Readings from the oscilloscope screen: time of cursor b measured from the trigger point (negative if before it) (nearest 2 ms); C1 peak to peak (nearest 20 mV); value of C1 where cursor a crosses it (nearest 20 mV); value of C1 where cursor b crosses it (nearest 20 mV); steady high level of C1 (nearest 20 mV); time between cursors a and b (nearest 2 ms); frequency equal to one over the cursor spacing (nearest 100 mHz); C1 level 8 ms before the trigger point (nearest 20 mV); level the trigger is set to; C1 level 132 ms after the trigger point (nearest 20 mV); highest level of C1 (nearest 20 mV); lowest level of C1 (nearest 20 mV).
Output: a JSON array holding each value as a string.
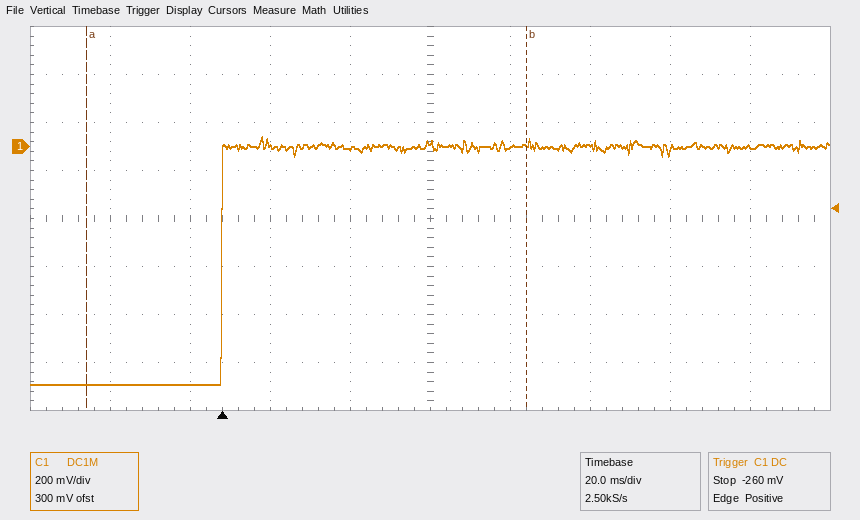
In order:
["+76 ms", "1.04 V", "-1.00 V", "20 mV", "0 mV", "110 ms", "9.1 Hz", "-1.00 V", "-260 mV", "0 mV", "40 mV", "-1.00 V"]
